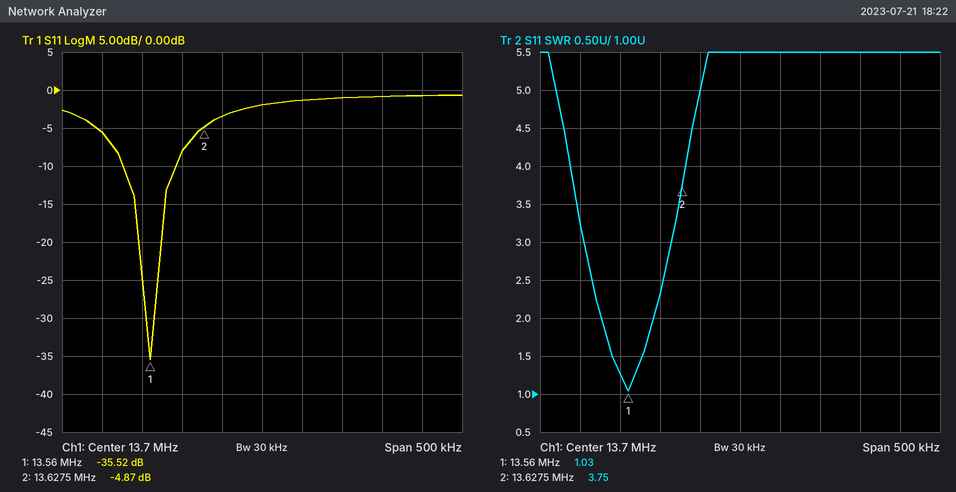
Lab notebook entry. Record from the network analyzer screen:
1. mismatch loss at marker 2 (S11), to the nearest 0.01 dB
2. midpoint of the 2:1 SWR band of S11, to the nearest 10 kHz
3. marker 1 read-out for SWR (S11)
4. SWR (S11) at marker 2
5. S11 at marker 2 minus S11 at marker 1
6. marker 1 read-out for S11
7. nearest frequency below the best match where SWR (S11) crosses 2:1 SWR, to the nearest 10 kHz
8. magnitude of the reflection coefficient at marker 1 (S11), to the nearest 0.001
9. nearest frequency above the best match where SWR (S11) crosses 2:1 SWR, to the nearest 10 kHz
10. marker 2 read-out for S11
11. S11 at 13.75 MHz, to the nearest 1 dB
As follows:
1.71 dB
13.56 MHz
1.03
3.75
30.65 dB
-35.52 dB
13.53 MHz
0.017
13.59 MHz
-4.87 dB
-1 dB
